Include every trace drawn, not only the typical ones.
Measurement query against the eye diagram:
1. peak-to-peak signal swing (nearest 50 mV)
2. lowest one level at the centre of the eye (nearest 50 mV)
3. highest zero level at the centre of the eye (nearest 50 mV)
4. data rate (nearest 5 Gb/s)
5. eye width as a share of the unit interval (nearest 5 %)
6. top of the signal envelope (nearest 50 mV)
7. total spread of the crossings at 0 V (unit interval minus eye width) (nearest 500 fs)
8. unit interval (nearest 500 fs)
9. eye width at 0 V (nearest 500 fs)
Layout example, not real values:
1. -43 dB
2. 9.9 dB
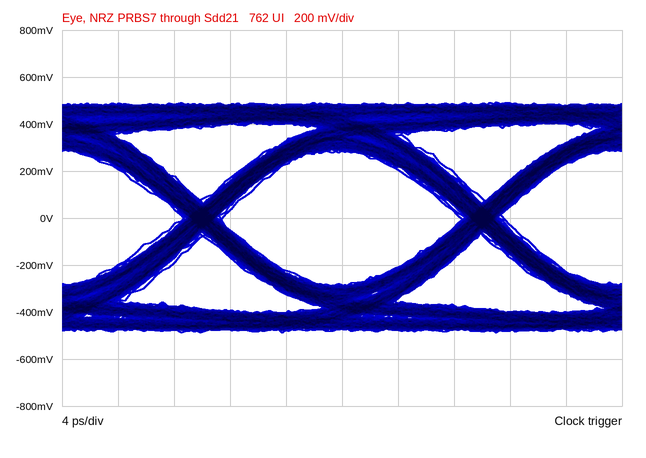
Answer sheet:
1. 1.00 V
2. 300 mV
3. -300 mV
4. 50 Gb/s
5. 85 %
6. 500 mV
7. 3.0 ps
8. 20.0 ps
9. 17.0 ps
